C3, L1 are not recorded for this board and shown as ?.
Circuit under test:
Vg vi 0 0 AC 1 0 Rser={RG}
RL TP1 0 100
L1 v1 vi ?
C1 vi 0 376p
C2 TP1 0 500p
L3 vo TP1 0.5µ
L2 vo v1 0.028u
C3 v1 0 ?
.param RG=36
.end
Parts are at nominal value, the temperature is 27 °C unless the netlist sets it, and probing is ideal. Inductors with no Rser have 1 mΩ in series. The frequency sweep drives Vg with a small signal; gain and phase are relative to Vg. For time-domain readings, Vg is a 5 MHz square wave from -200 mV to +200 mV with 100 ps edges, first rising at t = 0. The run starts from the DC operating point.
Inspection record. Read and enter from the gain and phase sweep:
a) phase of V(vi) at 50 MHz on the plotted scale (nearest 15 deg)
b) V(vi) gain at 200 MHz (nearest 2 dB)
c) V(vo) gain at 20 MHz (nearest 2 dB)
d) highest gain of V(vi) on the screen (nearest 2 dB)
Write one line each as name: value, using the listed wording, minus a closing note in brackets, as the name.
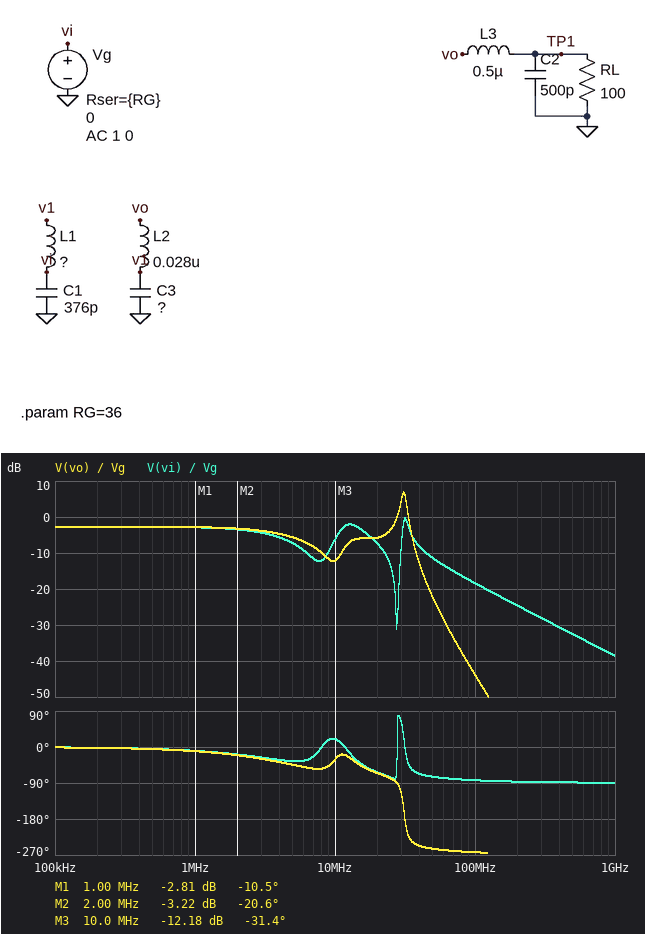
phase of V(vi) at 50 MHz on the plotted scale: -75 deg
V(vi) gain at 200 MHz: -24 dB
V(vo) gain at 20 MHz: -6 dB
highest gain of V(vi) on the screen: 0 dB
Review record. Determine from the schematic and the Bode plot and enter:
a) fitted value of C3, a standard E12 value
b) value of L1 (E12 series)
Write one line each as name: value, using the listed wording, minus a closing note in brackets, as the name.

fitted value of C3, a standard E12 value: 220 pF
value of L1: 220 nH
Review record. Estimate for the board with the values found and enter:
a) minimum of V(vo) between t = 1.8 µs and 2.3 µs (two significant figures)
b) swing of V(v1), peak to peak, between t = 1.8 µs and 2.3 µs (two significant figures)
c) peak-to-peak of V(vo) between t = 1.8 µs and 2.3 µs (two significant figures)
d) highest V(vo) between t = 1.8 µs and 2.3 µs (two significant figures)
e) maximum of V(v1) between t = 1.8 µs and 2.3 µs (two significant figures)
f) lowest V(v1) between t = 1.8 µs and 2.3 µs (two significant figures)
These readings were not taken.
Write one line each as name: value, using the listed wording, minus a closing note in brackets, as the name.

minimum of V(vo) between t = 1.8 µs and 2.3 µs: -170 mV
swing of V(v1), peak to peak, between t = 1.8 µs and 2.3 µs: 350 mV
peak-to-peak of V(vo) between t = 1.8 µs and 2.3 µs: 340 mV
highest V(vo) between t = 1.8 µs and 2.3 µs: 170 mV
maximum of V(v1) between t = 1.8 µs and 2.3 µs: 170 mV
lowest V(v1) between t = 1.8 µs and 2.3 µs: -170 mV
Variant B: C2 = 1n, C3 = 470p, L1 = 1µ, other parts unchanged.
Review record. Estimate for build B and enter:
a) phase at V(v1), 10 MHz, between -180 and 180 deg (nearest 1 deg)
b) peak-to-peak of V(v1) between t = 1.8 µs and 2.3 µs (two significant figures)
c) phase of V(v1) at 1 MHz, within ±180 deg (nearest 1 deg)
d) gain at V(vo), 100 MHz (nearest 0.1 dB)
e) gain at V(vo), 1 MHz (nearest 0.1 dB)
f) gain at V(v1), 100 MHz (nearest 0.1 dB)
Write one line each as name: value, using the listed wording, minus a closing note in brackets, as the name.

phase at V(v1), 10 MHz, between -180 and 180 deg: -36 deg
peak-to-peak of V(v1) between t = 1.8 µs and 2.3 µs: 340 mV
phase of V(v1) at 1 MHz, within ±180 deg: -20 deg
gain at V(vo), 100 MHz: -64.3 dB
gain at V(vo), 1 MHz: -2.9 dB
gain at V(v1), 100 MHz: -63.8 dB
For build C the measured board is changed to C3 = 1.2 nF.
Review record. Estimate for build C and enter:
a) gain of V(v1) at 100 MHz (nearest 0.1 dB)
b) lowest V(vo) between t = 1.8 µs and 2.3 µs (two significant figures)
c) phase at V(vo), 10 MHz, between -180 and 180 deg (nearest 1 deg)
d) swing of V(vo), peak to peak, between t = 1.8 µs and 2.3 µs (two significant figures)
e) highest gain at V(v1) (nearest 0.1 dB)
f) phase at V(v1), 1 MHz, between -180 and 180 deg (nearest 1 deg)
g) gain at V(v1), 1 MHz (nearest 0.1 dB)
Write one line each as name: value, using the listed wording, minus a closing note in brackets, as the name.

gain of V(v1) at 100 MHz: -58.6 dB
lowest V(vo) between t = 1.8 µs and 2.3 µs: -120 mV
phase at V(vo), 10 MHz, between -180 and 180 deg: -57 deg
swing of V(vo), peak to peak, between t = 1.8 µs and 2.3 µs: 230 mV
highest gain at V(v1): -2.7 dB
phase at V(v1), 1 MHz, between -180 and 180 deg: -19 deg
gain at V(v1), 1 MHz: -3.1 dB
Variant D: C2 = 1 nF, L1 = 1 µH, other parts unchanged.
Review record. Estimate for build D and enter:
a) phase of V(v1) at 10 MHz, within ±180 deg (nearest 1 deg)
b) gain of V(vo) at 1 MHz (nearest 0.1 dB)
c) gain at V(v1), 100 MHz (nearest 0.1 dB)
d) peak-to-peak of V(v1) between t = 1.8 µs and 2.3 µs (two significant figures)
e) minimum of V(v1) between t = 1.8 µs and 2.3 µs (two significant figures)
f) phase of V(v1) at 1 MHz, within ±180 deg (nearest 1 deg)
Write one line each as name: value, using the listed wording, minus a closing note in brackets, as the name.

phase of V(v1) at 10 MHz, within ±180 deg: -31 deg
gain of V(vo) at 1 MHz: -2.8 dB
gain at V(v1), 100 MHz: -57.1 dB
peak-to-peak of V(v1) between t = 1.8 µs and 2.3 µs: 230 mV
minimum of V(v1) between t = 1.8 µs and 2.3 µs: -110 mV
phase of V(v1) at 1 MHz, within ±180 deg: -17 deg
